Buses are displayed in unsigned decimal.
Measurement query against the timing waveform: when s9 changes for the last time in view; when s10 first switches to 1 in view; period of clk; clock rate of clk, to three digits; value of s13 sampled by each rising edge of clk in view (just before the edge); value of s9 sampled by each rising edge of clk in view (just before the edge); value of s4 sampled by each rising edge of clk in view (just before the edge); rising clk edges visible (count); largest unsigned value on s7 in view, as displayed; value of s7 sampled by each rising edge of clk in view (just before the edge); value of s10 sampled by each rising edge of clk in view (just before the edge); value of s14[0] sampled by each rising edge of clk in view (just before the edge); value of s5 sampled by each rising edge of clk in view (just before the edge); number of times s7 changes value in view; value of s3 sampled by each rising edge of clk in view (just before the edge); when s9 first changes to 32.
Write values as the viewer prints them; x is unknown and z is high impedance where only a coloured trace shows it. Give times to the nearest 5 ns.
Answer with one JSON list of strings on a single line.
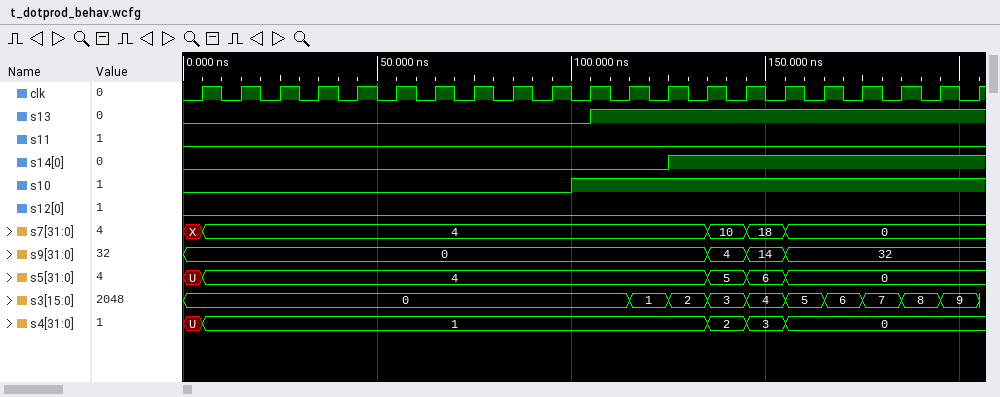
["155 ns", "100 ns", "10 ns", "100 MHz", "0 0 0 0 0 0 0 0 0 0 0 1 1 1 1 1 1 1 1 1 1", "0, 0, 0, 0, 0, 0, 0, 0, 0, 0, 0, 0, 0, 0, 4, 14, 32, 32, 32, 32, 32", "U, 1, 1, 1, 1, 1, 1, 1, 1, 1, 1, 1, 1, 1, 2, 3, 0, 0, 0, 0, 0", "21", "18", "X, 4, 4, 4, 4, 4, 4, 4, 4, 4, 4, 4, 4, 4, 10, 18, 0, 0, 0, 0, 0", "0 0 0 0 0 0 0 0 0 0 1 1 1 1 1 1 1 1 1 1 1", "0 0 0 0 0 0 0 0 0 0 0 0 0 1 1 1 1 1 1 1 1", "U, 4, 4, 4, 4, 4, 4, 4, 4, 4, 4, 4, 4, 4, 5, 6, 0, 0, 0, 0, 0", "4", "0, 0, 0, 0, 0, 0, 0, 0, 0, 0, 0, 0, 1, 2, 3, 4, 5, 6, 7, 8, 9", "155 ns"]
